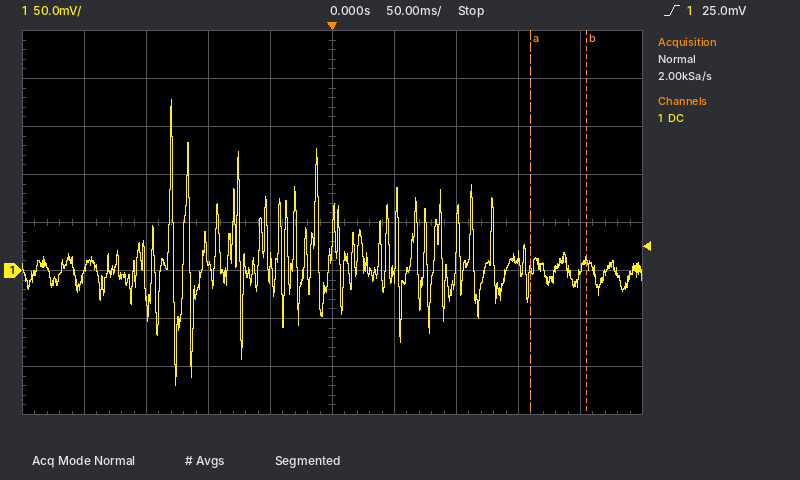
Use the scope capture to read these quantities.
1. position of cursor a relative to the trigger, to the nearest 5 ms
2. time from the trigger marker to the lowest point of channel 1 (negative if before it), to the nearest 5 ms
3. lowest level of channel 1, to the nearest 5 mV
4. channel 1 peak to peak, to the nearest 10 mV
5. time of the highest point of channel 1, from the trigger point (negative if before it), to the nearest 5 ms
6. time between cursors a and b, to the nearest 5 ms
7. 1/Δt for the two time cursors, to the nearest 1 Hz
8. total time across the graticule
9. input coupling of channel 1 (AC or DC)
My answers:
+160 ms
-125 ms
-120 mV
300 mV
-130 ms
45 ms
22 Hz
500 ms
DC
